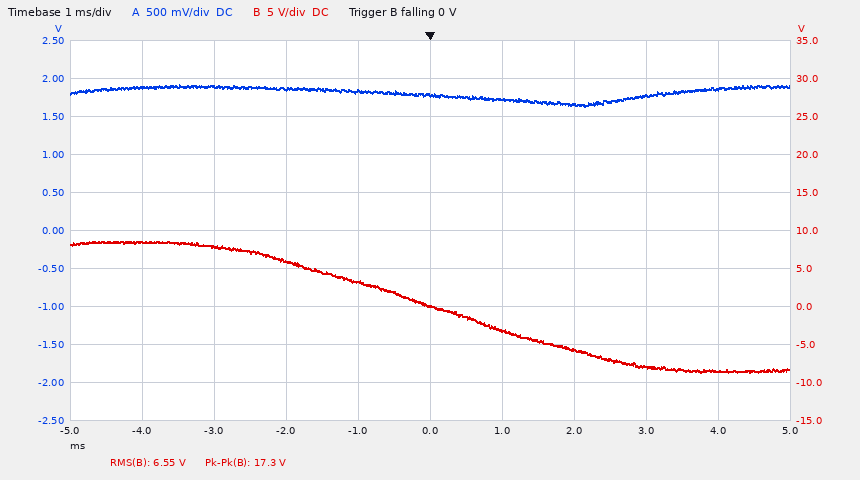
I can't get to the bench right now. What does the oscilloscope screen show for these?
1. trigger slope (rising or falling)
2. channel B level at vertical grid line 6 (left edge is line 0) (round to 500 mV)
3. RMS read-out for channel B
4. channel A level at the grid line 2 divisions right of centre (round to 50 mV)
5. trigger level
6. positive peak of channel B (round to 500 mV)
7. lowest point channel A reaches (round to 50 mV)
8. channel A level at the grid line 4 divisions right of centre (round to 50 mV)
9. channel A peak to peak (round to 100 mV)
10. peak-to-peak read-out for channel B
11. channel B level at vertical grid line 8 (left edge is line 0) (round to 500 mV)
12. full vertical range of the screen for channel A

falling
-3.0 V
6.55 V
1.65 V
0 V
8.5 V
1.65 V
1.85 V
300 mV
17.3 V
-8.0 V
5 V
